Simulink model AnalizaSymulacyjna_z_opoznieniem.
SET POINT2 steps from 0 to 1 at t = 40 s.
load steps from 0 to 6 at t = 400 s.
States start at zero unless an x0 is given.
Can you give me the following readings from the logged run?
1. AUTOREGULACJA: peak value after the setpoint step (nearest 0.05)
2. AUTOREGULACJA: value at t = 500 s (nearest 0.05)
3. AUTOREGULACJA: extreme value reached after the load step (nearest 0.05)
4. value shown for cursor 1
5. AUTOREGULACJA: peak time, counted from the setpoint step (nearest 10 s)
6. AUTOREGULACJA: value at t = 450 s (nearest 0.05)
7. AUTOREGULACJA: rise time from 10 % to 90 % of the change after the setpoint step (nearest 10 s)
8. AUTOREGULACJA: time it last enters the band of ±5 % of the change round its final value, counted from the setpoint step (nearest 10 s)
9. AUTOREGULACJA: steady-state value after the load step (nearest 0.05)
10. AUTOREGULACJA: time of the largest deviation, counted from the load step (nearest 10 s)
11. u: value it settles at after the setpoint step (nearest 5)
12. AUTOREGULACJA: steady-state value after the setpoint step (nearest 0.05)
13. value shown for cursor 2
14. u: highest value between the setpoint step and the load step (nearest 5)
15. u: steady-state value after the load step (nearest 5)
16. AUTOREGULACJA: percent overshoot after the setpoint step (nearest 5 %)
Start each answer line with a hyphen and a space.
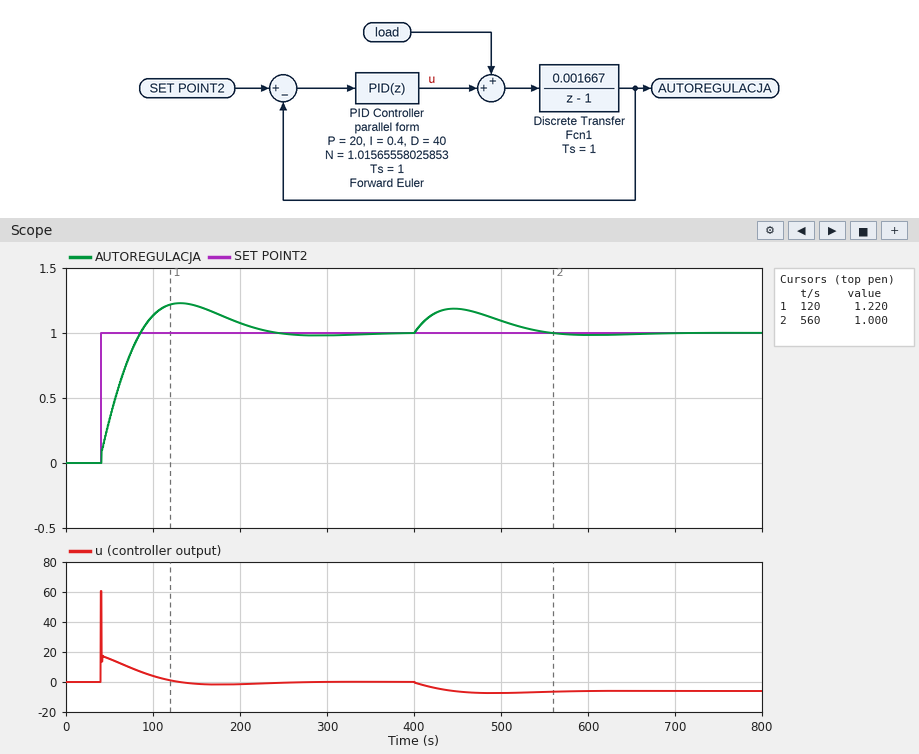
- 1.25
- 1.10
- 1.20
- 1.220
- 90 s
- 1.20
- 40 s
- 170 s
- 1.00
- 50 s
- 0
- 1.00
- 1.000
- 60
- -5
- 25 %
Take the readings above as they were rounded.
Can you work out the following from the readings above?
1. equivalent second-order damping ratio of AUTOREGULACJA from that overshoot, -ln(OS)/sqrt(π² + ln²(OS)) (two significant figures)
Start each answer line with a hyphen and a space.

- 0.40
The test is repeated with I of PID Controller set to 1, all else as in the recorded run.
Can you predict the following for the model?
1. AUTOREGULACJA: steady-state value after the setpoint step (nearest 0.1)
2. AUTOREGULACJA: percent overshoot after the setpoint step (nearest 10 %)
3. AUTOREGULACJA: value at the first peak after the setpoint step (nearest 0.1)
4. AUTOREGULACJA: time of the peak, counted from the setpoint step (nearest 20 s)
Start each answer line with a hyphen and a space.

- 1.0
- 40 %
- 1.4
- 60 s
